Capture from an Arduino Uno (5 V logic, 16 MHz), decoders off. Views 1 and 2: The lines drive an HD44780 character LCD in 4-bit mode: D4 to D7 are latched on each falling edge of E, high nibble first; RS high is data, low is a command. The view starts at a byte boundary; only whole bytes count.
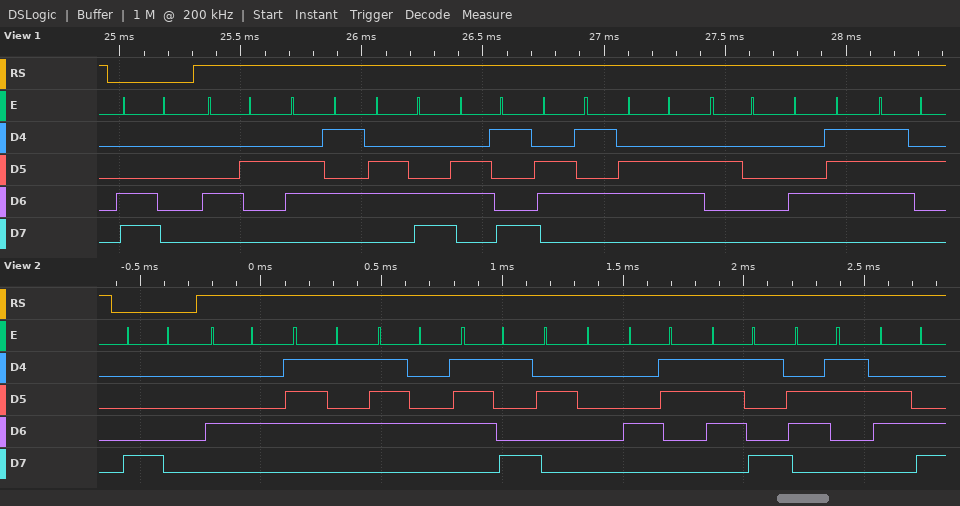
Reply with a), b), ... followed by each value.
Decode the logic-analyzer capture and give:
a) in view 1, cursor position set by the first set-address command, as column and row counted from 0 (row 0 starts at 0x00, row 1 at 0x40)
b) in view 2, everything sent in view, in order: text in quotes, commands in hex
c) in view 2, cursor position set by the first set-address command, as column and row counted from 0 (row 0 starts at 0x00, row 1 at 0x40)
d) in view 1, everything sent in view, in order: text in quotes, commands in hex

a) column 0, row 1
b) 0x80 "Duty Cycl"
c) column 0, row 0
d) 0xC0 "Belief Gr"
